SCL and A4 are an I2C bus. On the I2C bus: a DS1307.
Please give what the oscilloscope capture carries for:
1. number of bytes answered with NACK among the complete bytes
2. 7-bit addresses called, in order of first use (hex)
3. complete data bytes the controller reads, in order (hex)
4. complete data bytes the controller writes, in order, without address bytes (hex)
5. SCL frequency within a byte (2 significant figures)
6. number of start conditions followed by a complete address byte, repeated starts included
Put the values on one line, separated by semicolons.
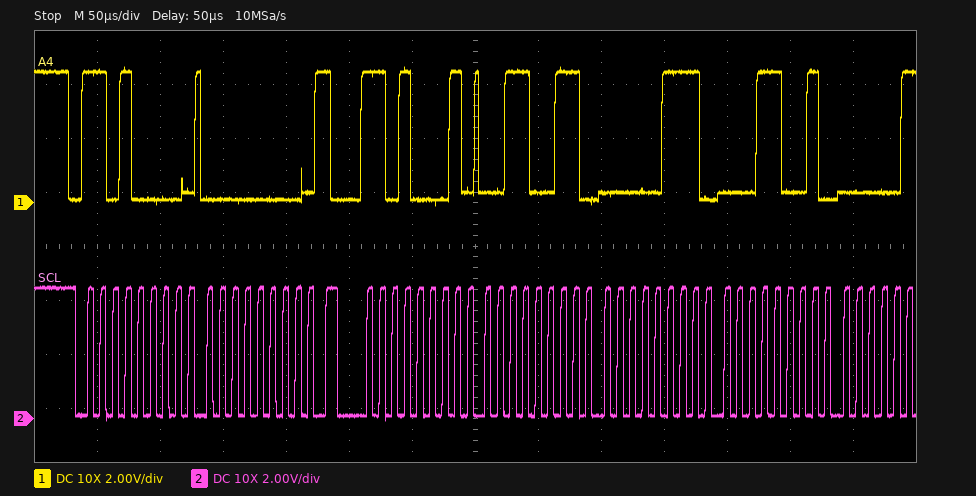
0; 0x68; 33 07 19; 00; 100 kHz; 2
